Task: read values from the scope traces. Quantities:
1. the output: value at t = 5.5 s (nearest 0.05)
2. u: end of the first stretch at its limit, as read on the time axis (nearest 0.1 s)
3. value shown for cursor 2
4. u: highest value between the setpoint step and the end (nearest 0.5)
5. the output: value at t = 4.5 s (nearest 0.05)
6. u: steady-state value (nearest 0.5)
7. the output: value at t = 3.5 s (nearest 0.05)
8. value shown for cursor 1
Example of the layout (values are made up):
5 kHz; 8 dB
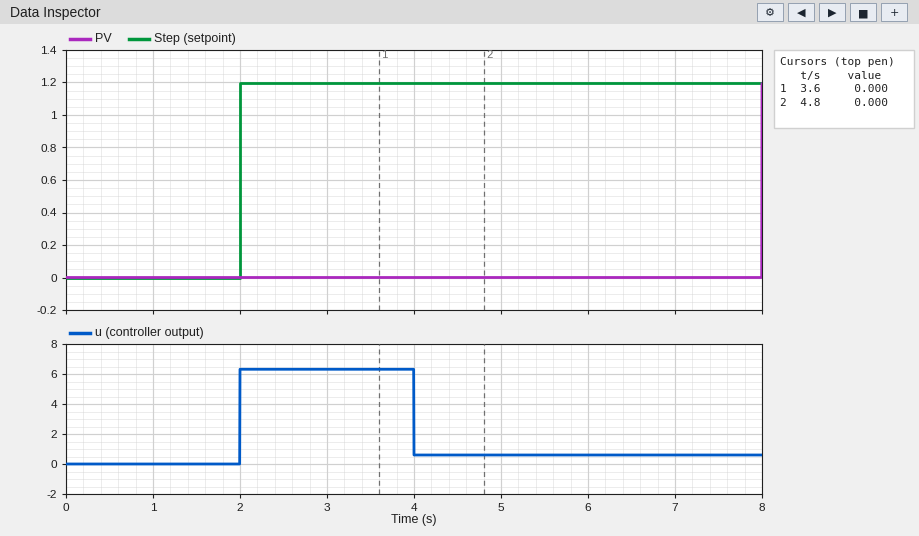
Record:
0.00; 4.0 s; 0.000; 6.5; 0.00; 0.5; 0.00; 0.000
